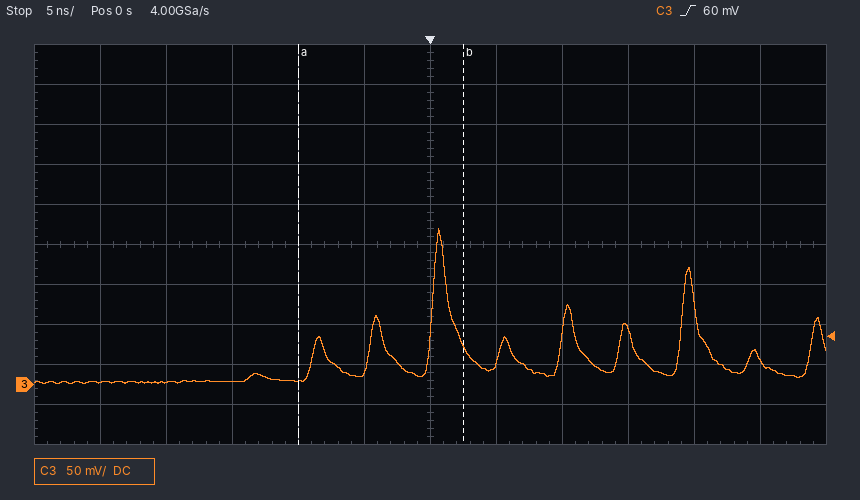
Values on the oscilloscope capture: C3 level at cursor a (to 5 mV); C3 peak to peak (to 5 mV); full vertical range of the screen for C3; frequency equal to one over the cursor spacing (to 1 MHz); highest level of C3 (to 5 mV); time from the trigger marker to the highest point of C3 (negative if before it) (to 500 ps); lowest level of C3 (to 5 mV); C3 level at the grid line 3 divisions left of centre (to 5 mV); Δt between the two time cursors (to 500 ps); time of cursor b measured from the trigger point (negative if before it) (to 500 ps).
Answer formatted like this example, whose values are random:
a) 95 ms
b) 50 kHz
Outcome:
a) 5 mV
b) 195 mV
c) 500 mV
d) 80 MHz
e) 195 mV
f) +500 ps
g) 0 mV
h) 5 mV
i) 12.5 ns
j) +2.5 ns
